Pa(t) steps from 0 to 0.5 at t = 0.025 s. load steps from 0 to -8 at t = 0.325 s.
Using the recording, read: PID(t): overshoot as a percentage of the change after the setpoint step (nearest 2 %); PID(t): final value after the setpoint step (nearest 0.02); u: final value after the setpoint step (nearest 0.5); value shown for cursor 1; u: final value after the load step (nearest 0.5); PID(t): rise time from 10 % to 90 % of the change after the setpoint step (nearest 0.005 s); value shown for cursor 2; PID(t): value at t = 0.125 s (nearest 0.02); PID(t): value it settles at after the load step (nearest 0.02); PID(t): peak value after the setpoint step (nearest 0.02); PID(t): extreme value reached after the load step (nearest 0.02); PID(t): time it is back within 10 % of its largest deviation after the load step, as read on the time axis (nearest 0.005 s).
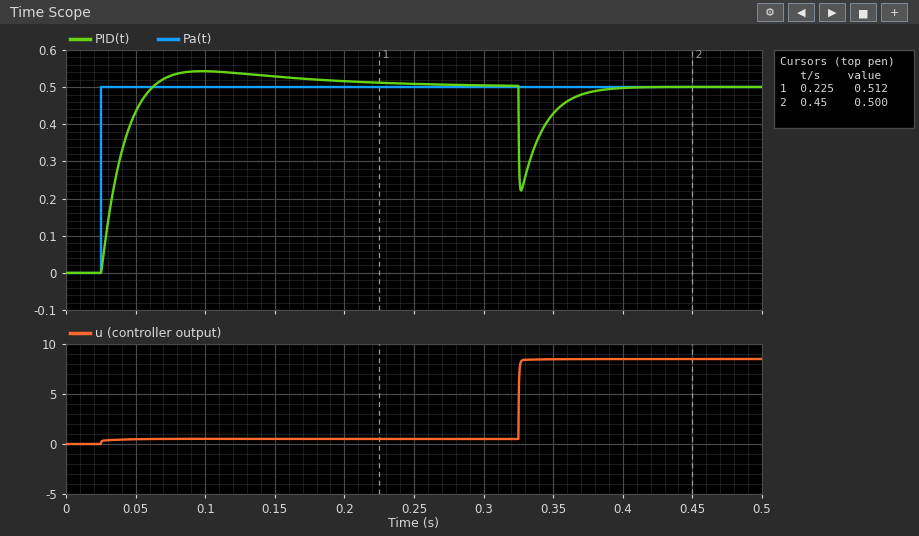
8 %
0.50
0.5
0.512
8.5
0.025 s
0.500
0.54
0.50
0.54
0.22
0.365 s
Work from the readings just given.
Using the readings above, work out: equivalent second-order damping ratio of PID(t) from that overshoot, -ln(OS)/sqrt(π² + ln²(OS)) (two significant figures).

0.63
